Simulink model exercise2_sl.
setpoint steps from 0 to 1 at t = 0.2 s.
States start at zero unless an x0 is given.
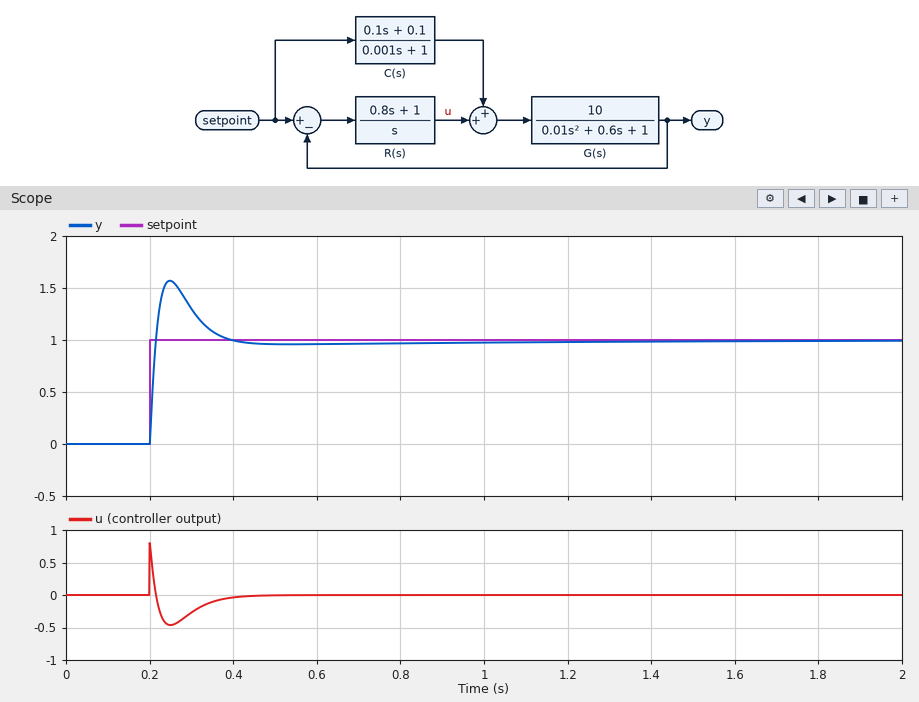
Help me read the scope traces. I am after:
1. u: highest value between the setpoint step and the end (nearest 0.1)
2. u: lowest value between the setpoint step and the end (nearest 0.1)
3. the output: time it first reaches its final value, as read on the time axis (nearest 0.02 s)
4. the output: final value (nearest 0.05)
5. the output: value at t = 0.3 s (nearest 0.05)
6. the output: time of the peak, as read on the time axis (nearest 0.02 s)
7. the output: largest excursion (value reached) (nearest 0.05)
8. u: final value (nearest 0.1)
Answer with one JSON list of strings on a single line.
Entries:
["0.8", "-0.5", "0.22 s", "1.00", "1.30", "0.24 s", "1.55", "0.0"]
